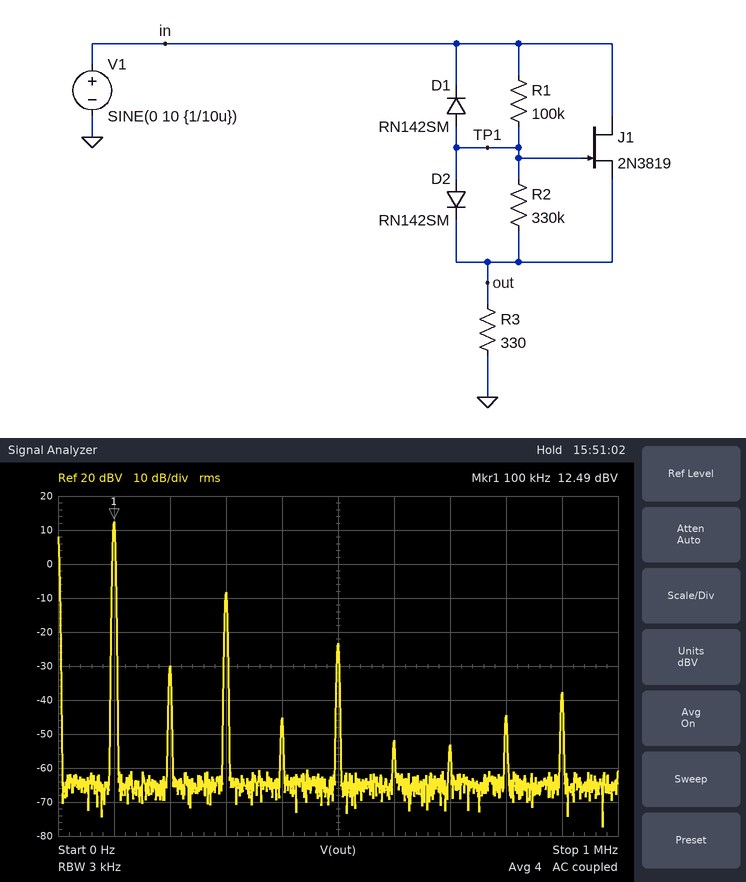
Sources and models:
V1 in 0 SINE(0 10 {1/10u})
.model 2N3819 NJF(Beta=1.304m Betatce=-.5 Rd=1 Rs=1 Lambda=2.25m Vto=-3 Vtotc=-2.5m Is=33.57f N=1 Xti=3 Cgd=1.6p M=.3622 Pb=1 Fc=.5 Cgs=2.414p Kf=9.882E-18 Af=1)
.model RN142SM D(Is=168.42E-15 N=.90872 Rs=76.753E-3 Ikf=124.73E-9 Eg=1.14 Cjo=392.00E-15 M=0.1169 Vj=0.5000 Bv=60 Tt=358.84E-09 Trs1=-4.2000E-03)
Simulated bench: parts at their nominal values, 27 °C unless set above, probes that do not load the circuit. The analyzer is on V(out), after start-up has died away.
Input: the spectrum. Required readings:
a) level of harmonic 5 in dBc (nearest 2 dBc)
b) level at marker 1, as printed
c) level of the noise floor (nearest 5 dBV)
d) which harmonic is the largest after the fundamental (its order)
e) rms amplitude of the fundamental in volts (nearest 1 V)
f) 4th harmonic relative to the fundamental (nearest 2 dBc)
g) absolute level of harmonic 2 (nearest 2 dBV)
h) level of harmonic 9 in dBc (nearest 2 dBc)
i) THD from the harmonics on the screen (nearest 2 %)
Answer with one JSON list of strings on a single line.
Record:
["-36 dBc", "12.49 dBV", "-65 dBV", "3", "4 V", "-58 dBc", "-30 dBV", "-50 dBc", "10 %"]
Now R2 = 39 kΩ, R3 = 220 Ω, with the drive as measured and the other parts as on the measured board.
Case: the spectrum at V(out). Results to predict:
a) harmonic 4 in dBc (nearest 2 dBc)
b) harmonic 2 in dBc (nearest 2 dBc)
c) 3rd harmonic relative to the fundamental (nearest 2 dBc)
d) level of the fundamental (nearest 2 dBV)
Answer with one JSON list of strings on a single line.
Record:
["-56 dBc", "-48 dBc", "-16 dBc", "10 dBV"]
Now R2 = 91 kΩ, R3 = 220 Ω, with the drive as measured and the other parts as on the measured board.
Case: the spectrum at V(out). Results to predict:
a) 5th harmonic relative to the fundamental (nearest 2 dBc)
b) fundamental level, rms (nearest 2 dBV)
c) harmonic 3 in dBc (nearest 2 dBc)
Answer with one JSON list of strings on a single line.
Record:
["-40 dBc", "10 dBV", "-16 dBc"]
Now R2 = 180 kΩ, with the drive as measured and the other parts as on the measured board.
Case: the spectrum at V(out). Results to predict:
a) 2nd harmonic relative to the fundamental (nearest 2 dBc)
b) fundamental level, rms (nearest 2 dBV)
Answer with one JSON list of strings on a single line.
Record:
["-50 dBc", "12 dBV"]
